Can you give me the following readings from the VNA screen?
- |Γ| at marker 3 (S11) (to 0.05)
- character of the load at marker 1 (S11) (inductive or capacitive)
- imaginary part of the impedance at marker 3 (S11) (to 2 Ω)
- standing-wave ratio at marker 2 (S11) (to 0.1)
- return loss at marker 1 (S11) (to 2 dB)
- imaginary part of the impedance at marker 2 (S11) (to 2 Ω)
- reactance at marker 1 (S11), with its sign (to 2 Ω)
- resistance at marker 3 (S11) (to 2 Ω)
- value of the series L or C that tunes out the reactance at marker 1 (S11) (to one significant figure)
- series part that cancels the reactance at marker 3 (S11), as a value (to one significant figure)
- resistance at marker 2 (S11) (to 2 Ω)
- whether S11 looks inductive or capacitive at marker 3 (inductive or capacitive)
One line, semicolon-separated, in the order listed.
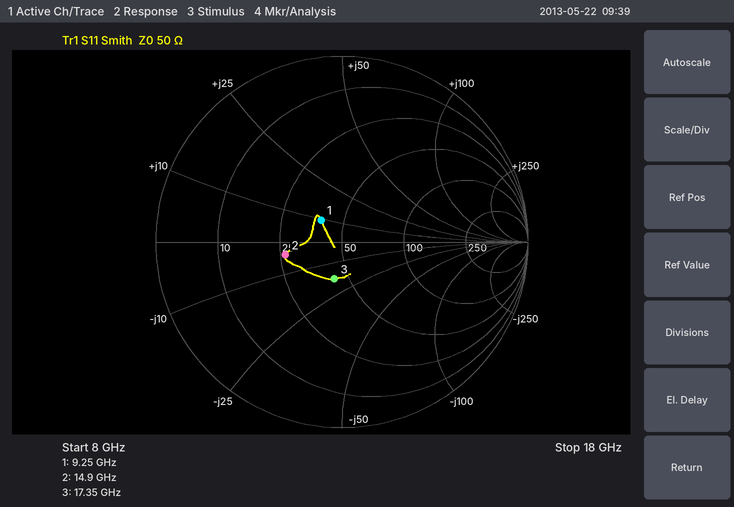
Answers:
0.20; inductive; -18 Ω; 1.9; 16 dB; -4 Ω; +10 Ω; 42 Ω; 2 pF; 200 pH; 26 Ω; capacitive
